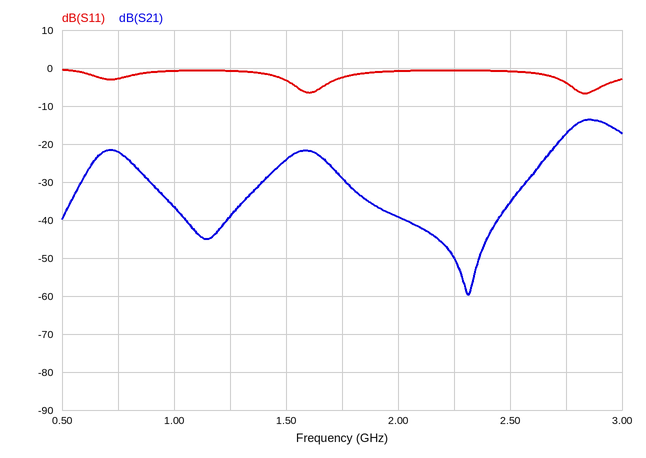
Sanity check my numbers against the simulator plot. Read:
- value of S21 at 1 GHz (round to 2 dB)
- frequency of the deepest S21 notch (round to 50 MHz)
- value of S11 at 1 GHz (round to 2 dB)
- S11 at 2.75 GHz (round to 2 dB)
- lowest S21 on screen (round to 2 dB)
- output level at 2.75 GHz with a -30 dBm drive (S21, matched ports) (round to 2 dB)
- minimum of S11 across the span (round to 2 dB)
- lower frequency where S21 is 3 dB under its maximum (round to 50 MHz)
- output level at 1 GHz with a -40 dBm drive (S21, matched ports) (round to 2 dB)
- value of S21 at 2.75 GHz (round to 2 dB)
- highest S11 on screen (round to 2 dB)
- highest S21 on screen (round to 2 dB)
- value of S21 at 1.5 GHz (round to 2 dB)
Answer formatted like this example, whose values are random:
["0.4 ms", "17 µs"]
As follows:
["-36 dB", "2.30 GHz", "0 dB", "-4 dB", "-60 dB", "-48 dBm", "-6 dB", "2.75 GHz", "-76 dBm", "-18 dB", "0 dB", "-14 dB", "-24 dB"]
